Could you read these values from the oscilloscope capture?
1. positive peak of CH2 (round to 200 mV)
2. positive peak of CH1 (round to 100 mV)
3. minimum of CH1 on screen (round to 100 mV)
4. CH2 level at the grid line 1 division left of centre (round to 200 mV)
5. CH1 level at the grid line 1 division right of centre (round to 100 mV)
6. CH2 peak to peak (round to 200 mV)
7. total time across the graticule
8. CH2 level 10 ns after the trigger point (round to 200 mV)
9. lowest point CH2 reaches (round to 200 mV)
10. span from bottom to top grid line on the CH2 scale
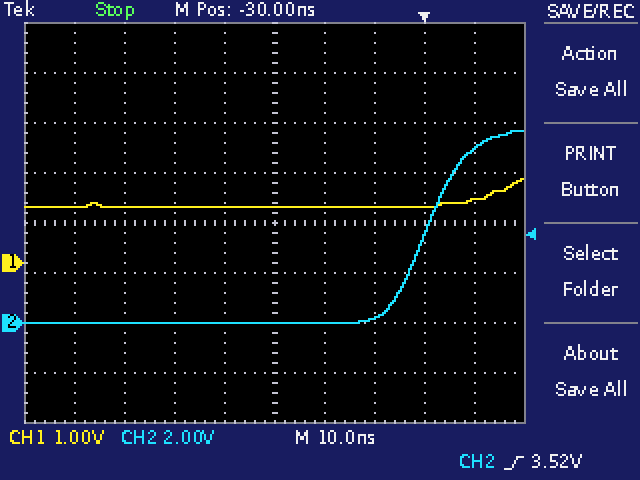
7.6 V
1.7 V
1.1 V
0.0 V
1.1 V
7.6 V
100 ns
7.0 V
0.0 V
16 V
